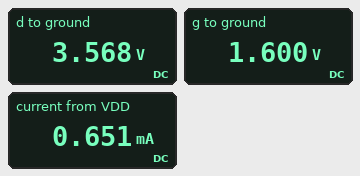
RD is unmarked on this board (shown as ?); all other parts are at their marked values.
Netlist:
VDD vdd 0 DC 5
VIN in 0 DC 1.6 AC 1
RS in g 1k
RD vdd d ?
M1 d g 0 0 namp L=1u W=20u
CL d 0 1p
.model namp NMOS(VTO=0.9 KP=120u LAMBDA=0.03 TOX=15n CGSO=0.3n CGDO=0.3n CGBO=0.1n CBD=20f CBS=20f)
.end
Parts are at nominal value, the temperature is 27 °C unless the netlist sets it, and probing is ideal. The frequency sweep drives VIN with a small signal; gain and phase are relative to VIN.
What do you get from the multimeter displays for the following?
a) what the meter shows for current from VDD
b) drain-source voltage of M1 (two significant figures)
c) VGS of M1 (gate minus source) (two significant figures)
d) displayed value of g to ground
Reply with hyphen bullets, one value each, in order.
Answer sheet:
- 0.651 mA
- 3.6 V
- 1.6 V
- 1.600 V
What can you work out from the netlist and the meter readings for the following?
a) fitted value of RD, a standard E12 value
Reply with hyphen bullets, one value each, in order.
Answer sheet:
- 2.2 kΩ
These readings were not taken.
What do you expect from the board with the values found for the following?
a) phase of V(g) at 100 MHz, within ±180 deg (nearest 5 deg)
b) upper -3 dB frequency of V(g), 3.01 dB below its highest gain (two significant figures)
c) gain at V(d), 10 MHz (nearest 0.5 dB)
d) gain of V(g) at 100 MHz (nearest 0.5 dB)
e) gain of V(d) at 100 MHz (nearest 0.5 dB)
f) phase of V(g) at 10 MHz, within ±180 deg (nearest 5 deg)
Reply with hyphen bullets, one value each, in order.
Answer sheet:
- 0 deg
- 3.7 GHz
- 12.0 dB
- 0 dB
- 7.5 dB
- 0 deg
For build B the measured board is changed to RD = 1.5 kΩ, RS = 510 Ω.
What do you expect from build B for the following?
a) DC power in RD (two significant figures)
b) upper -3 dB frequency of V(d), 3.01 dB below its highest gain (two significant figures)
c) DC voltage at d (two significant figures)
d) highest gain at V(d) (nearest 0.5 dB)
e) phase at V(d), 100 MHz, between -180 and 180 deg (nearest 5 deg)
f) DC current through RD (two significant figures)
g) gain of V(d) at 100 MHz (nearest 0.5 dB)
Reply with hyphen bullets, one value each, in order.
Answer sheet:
- 650 µW
- 110 MHz
- 4.0 V
- 9.0 dB
- 135 deg
- 660 µA
- 6.0 dB
